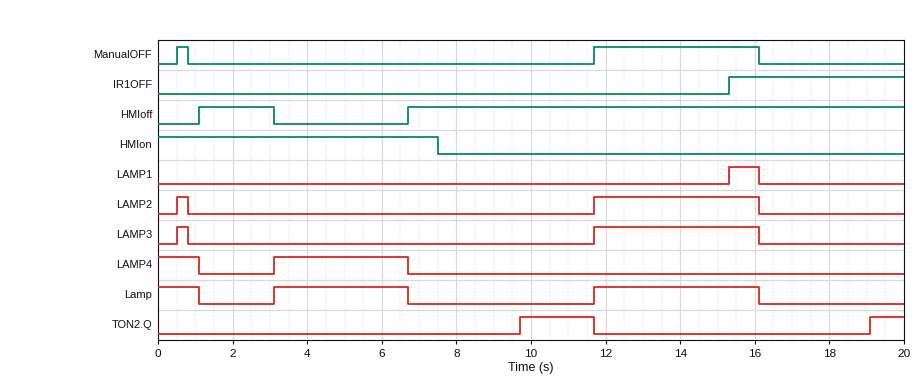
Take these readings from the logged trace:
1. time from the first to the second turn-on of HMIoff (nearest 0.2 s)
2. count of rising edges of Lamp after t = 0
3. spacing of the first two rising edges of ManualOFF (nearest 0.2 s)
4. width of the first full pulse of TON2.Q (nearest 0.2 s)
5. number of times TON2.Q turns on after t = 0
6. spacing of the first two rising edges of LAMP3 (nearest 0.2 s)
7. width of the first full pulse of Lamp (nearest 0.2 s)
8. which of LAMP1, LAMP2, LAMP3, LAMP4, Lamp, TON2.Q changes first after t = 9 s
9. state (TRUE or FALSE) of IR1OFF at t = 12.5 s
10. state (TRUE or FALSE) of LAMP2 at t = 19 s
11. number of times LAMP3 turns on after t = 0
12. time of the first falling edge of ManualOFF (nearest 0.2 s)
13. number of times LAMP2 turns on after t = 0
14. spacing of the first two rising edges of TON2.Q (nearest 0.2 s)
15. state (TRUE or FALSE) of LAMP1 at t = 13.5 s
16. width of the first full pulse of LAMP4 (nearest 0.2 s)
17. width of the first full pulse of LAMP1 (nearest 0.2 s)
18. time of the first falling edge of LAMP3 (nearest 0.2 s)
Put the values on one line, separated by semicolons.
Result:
5.6 s; 2; 11.2 s; 2.0 s; 2; 11.2 s; 3.6 s; TON2.Q; FALSE; FALSE; 2; 0.8 s; 2; 9.4 s; FALSE; 3.6 s; 0.8 s; 0.8 s
